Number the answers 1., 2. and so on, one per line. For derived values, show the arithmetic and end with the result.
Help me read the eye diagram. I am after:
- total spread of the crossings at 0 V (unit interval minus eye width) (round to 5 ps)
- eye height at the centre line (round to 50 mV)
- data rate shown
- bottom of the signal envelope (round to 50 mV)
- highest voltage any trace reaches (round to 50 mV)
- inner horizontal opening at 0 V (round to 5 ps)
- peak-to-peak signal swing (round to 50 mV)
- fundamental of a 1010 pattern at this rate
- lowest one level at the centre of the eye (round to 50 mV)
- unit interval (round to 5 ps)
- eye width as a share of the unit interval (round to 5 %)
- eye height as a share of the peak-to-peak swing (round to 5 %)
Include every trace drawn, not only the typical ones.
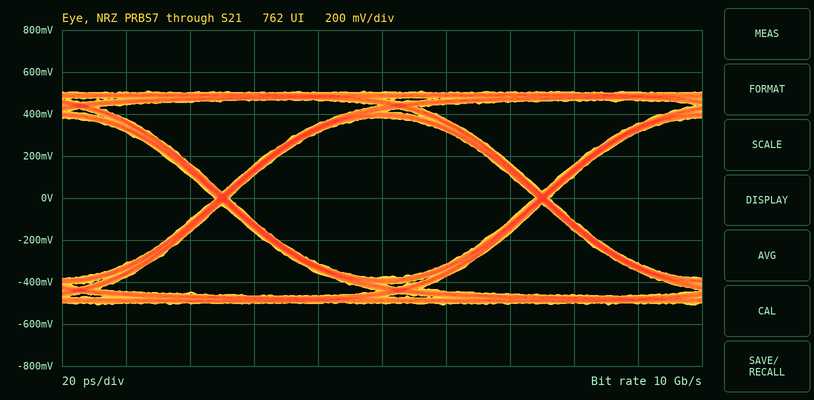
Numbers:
1. 5 ps
2. 750 mV
3. 10 Gb/s
4. -500 mV
5. 500 mV
6. 95 ps
7. 1.00 V
8. 5 GHz
9. 400 mV
10. 100 ps
11. 95 ps / 100 ps ≈ 95 %
12. 750 mV / 1.00 V ≈ 75 %
